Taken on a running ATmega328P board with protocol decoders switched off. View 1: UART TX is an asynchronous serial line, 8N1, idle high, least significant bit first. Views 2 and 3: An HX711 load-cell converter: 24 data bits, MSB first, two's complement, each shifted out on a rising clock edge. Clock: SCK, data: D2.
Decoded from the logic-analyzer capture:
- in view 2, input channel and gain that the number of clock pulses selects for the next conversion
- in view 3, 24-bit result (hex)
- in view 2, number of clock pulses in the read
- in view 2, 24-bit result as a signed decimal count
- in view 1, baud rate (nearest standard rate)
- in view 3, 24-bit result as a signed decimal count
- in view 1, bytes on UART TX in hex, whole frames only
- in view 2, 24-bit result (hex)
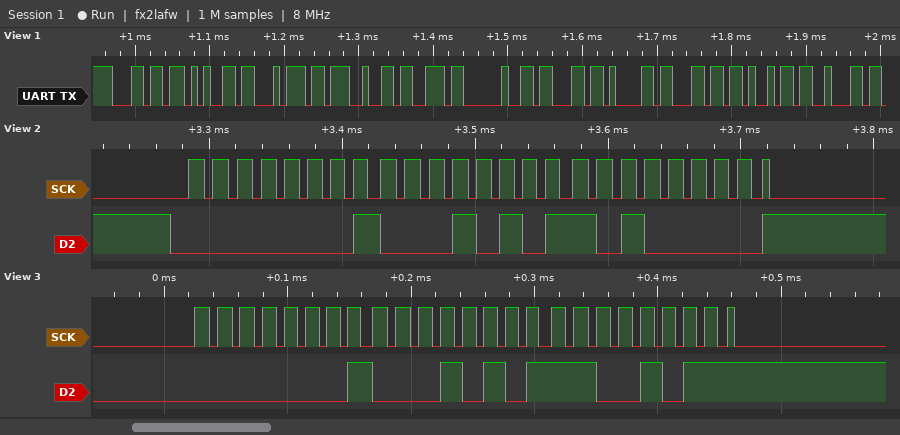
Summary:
channel A, gain 128
0x0115CB
25
71072
115200 baud
71115
0x6C 0x65 0x74 0x27 0x73 0x20 0x63 0x61 0x6C 0x69 0x62
0x0115A0
